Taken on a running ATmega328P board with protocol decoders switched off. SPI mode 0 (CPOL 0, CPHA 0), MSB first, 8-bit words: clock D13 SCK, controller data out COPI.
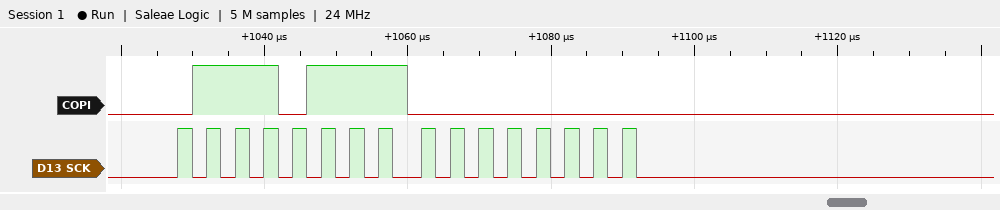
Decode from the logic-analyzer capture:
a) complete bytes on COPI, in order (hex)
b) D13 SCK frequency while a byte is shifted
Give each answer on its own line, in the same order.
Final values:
77 00
250 kHz
